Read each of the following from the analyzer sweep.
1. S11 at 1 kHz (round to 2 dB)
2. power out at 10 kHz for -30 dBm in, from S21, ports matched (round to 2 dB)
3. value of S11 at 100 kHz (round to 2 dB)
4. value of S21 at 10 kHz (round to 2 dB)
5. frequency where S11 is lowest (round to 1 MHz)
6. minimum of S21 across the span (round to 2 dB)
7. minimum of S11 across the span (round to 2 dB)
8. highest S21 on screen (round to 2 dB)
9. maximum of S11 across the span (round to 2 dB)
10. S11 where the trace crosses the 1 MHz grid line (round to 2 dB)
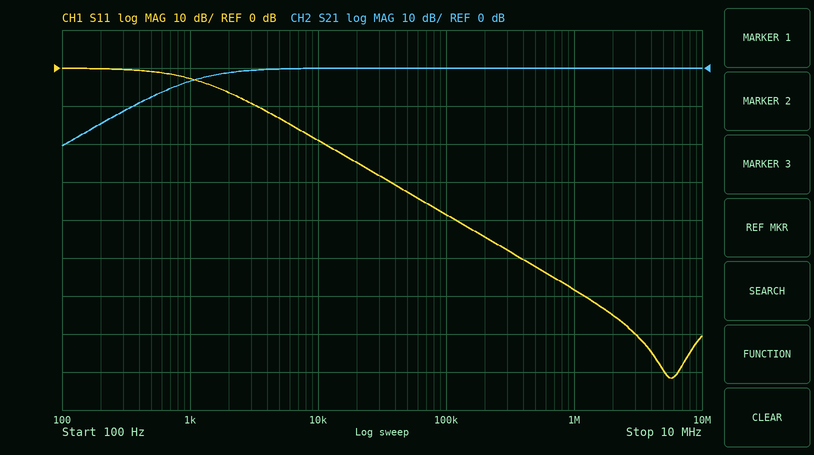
-2 dB
-30 dBm
-38 dB
0 dB
6 MHz
-20 dB
-82 dB
0 dB
0 dB
-58 dB
